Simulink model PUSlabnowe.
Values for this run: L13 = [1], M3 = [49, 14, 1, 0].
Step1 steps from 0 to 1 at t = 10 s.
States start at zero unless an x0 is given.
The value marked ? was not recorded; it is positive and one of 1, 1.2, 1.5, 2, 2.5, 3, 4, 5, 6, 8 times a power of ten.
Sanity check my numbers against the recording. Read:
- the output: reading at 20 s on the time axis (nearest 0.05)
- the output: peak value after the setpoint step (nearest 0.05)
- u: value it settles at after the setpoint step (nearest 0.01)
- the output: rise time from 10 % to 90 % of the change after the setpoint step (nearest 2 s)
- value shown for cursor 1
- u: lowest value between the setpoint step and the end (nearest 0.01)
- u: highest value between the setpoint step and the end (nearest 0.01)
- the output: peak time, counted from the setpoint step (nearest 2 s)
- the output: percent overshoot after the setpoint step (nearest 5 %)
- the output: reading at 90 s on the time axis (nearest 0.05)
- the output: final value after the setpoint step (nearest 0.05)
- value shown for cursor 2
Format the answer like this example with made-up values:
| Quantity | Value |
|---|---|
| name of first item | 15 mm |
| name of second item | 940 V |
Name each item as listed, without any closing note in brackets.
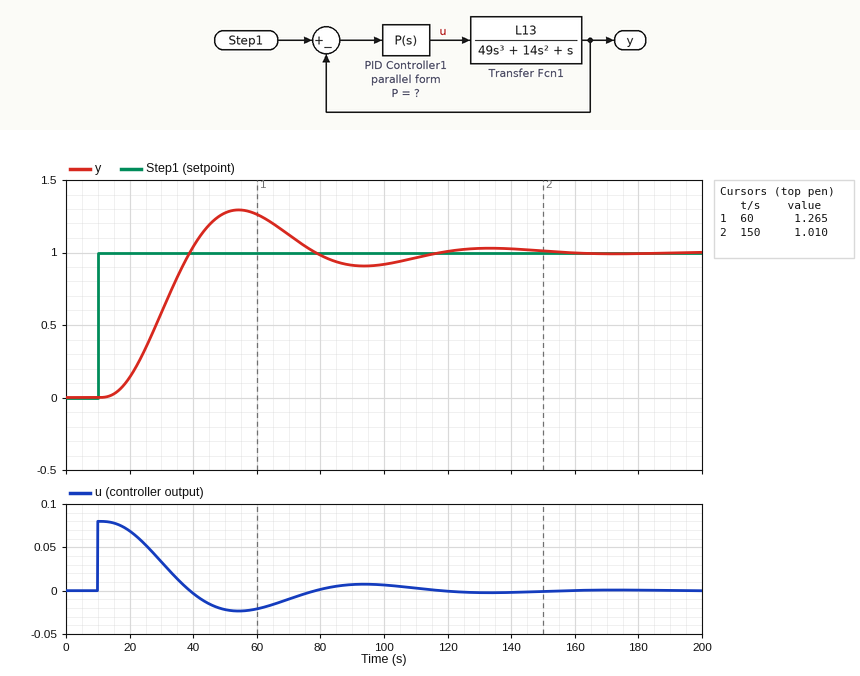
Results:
| Quantity | Value |
|---|---|
| the output: reading at 20 s on the time axis | 0.15 |
| the output: peak value after the setpoint step | 1.30 |
| u: value it settles at after the setpoint step | 0.00 |
| the output: rise time from 10 % to 90 % of the change after the setpoint step | 18 s |
| value shown for cursor 1 | 1.265 |
| u: lowest value between the setpoint step and the end | -0.02 |
| u: highest value between the setpoint step and the end | 0.08 |
| the output: peak time, counted from the setpoint step | 44 s |
| the output: percent overshoot after the setpoint step | 30 % |
| the output: reading at 90 s on the time axis | 0.90 |
| the output: final value after the setpoint step | 1.00 |
| value shown for cursor 2 | 1.010 |
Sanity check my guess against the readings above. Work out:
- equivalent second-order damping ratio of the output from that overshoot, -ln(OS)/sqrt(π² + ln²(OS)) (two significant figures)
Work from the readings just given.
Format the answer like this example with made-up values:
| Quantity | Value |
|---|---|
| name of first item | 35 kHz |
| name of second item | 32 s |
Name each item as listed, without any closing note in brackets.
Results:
| Quantity | Value |
|---|---|
| equivalent second-order damping ratio of the output from that overshoot, -ln(OS)/sqrt(π² + ln²(OS)) | 0.36 |
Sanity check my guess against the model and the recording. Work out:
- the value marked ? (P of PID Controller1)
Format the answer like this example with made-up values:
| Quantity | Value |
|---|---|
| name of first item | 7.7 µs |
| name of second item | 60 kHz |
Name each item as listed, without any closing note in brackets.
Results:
| Quantity | Value |
|---|---|
| the value marked ? | 0.08 |
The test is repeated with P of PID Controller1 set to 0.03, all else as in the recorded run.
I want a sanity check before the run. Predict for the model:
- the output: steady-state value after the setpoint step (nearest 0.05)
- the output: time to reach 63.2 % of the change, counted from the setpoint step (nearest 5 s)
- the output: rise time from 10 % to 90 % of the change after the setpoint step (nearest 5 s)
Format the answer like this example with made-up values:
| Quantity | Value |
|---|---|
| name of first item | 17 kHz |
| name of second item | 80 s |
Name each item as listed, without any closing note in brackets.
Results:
| Quantity | Value |
|---|---|
| the output: steady-state value after the setpoint step | 1.00 |
| the output: time to reach 63.2 % of the change, counted from the setpoint step | 40 s |
| the output: rise time from 10 % to 90 % of the change after the setpoint step | 45 s |
